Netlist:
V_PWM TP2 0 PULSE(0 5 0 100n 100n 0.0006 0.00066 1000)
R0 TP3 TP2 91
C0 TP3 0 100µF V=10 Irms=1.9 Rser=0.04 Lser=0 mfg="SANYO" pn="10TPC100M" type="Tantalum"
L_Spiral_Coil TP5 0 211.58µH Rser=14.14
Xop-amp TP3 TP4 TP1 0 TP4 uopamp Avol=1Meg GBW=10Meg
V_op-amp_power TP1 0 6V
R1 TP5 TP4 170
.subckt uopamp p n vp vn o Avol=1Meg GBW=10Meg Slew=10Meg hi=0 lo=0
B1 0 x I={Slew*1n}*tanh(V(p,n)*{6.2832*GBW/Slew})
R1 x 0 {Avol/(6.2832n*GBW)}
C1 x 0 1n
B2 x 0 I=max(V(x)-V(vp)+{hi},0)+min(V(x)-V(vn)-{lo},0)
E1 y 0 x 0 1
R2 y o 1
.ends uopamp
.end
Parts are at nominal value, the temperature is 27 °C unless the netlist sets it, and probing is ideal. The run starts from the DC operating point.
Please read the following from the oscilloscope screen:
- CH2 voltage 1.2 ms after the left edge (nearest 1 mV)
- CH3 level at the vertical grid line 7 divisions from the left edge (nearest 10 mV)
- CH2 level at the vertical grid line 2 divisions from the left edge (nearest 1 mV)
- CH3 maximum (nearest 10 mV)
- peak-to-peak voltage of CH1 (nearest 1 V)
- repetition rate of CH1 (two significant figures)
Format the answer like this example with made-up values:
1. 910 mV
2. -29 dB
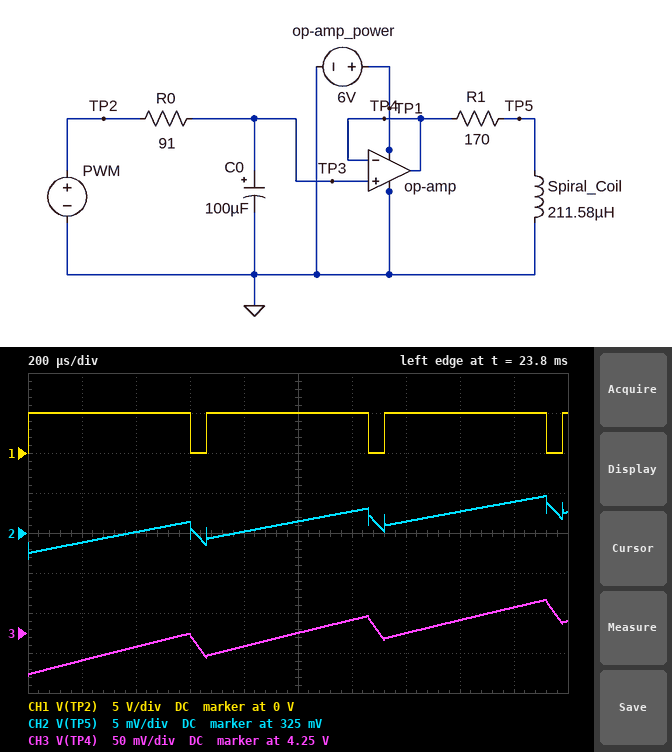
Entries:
1. 328 mV
2. 4.25 V
3. 325 mV
4. 4.29 V
5. 5 V
6. 1.5 kHz
